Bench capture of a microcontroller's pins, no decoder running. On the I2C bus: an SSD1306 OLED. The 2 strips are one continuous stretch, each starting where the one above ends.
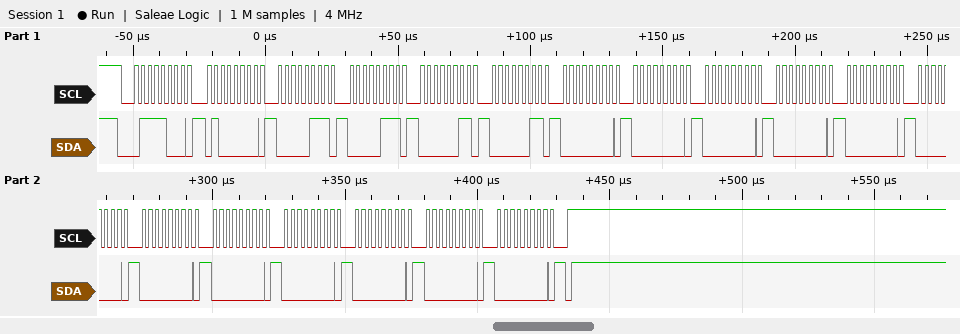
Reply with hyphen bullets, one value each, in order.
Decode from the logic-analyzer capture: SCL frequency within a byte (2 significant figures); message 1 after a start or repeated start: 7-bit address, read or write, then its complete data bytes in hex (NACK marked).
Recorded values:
- 400 kHz
- 0x3C write: 40 07 07 03 03 00 00 00 00 00 00 00 00 00 00 00 00
